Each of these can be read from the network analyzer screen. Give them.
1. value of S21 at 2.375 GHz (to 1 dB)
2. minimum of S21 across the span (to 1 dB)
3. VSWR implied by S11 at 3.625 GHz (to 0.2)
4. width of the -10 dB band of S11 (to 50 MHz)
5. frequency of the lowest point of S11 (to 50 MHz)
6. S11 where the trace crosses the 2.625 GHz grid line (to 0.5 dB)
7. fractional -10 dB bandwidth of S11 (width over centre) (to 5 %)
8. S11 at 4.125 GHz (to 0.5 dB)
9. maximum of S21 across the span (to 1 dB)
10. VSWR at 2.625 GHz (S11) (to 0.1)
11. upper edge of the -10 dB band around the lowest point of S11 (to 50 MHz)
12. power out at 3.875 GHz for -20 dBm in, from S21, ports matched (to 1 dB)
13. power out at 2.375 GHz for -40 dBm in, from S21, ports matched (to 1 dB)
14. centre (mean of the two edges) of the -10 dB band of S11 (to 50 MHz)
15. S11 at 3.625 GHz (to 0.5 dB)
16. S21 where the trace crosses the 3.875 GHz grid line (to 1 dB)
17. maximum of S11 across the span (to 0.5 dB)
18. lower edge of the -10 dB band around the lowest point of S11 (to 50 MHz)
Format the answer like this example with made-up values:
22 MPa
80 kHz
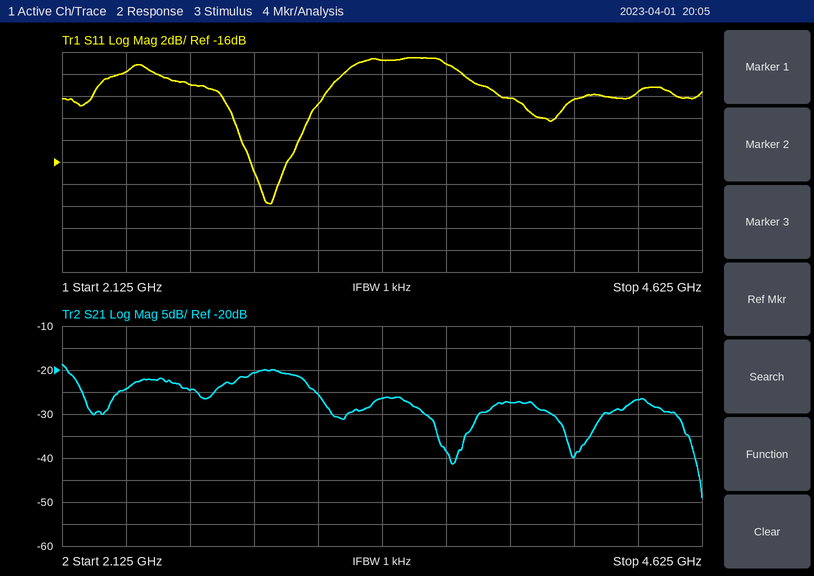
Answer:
-24 dB
-49 dB
2.6
400 MHz
2.95 GHz
-9.0 dB
15 %
-10.5 dB
-19 dB
2.1
3.15 GHz
-47 dBm
-64 dBm
2.95 GHz
-7.0 dB
-27 dB
-6.5 dB
2.75 GHz
